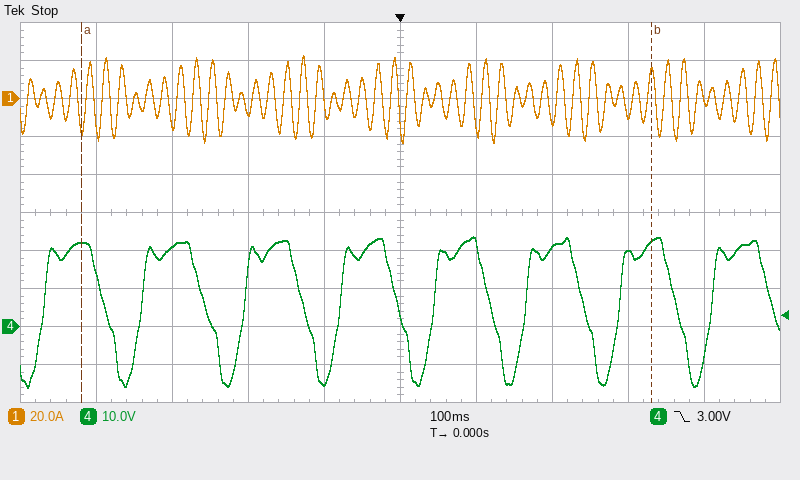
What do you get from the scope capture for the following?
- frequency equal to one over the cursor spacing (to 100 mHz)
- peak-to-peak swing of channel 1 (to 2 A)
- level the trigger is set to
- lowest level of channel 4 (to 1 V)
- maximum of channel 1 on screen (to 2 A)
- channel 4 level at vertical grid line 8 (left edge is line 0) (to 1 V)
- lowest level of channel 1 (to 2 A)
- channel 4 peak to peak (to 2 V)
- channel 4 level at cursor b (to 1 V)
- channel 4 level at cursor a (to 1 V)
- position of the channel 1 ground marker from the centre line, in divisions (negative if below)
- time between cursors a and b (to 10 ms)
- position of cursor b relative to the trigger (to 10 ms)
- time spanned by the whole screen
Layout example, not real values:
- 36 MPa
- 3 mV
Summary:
- 1.3 Hz
- 46 A
- 3.00 V
- -16 V
- 22 A
- 19 V
- -24 A
- 40 V
- 22 V
- 22 V
- +3.0 div
- 750 ms
- +330 ms
- 1 s
